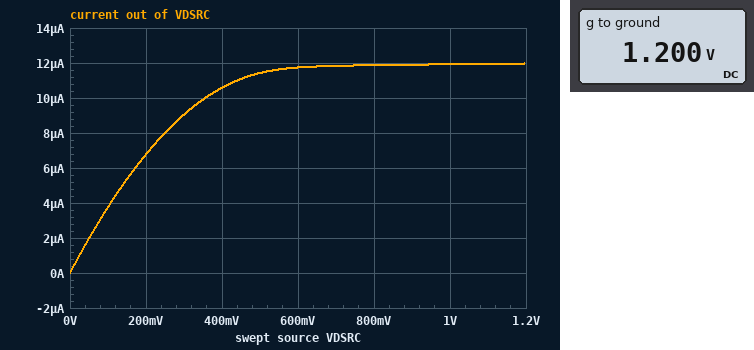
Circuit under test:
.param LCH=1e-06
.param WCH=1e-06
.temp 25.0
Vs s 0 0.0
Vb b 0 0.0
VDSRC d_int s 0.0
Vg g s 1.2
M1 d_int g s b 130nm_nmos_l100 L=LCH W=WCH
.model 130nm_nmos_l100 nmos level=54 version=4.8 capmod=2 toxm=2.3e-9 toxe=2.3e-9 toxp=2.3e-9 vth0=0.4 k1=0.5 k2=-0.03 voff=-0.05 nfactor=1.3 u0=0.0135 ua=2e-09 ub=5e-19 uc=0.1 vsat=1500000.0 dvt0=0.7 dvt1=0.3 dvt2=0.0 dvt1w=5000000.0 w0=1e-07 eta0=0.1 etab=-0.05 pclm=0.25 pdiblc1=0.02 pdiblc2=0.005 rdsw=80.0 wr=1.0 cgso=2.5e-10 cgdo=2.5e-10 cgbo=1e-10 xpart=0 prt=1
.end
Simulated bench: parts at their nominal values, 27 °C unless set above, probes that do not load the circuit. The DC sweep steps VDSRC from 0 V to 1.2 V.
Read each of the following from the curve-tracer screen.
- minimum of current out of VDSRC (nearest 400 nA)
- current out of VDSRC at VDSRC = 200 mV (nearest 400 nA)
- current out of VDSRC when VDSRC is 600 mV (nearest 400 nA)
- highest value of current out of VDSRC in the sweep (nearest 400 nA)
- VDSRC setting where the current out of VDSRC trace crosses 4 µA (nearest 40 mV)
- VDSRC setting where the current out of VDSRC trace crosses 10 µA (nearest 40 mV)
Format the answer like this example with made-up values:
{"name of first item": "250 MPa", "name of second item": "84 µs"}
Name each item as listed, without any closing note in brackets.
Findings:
{"minimum of current out of VDSRC": "0 A", "current out of VDSRC at VDSRC = 200 mV": "6.8 µA", "current out of VDSRC when VDSRC is 600 mV": "11.6 µA", "highest value of current out of VDSRC in the sweep": "12.0 µA", "VDSRC setting where the current out of VDSRC trace crosses 4 µA": "120 mV", "VDSRC setting where the current out of VDSRC trace crosses 10 µA": "360 mV"}
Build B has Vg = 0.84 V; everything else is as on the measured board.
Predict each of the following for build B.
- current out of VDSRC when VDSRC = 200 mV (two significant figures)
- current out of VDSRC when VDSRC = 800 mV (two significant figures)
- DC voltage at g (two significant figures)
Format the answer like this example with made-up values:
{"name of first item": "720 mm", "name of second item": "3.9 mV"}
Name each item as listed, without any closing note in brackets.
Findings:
{"current out of VDSRC when VDSRC = 200 mV": "2.3 µA", "current out of VDSRC when VDSRC = 800 mV": "2.6 µA", "DC voltage at g": "840 mV"}
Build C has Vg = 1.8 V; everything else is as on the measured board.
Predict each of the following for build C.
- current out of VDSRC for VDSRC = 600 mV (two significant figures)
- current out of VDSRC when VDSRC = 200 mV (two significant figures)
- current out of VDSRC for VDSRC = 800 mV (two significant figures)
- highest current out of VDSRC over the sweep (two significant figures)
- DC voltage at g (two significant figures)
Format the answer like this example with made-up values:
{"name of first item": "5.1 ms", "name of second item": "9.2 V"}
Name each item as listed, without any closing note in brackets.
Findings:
{"current out of VDSRC for VDSRC = 600 mV": "28 µA", "current out of VDSRC when VDSRC = 200 mV": "12 µA", "current out of VDSRC for VDSRC = 800 mV": "32 µA", "highest current out of VDSRC over the sweep": "35 µA", "DC voltage at g": "1.8 V"}
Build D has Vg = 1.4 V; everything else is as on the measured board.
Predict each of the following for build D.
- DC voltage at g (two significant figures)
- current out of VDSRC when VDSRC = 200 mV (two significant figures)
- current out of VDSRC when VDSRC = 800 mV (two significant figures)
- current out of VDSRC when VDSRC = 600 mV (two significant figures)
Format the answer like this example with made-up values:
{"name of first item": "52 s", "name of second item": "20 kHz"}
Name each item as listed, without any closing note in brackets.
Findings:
{"DC voltage at g": "1.4 V", "current out of VDSRC when VDSRC = 200 mV": "8.7 µA", "current out of VDSRC when VDSRC = 800 mV": "19 µA", "current out of VDSRC when VDSRC = 600 mV": "18 µA"}
